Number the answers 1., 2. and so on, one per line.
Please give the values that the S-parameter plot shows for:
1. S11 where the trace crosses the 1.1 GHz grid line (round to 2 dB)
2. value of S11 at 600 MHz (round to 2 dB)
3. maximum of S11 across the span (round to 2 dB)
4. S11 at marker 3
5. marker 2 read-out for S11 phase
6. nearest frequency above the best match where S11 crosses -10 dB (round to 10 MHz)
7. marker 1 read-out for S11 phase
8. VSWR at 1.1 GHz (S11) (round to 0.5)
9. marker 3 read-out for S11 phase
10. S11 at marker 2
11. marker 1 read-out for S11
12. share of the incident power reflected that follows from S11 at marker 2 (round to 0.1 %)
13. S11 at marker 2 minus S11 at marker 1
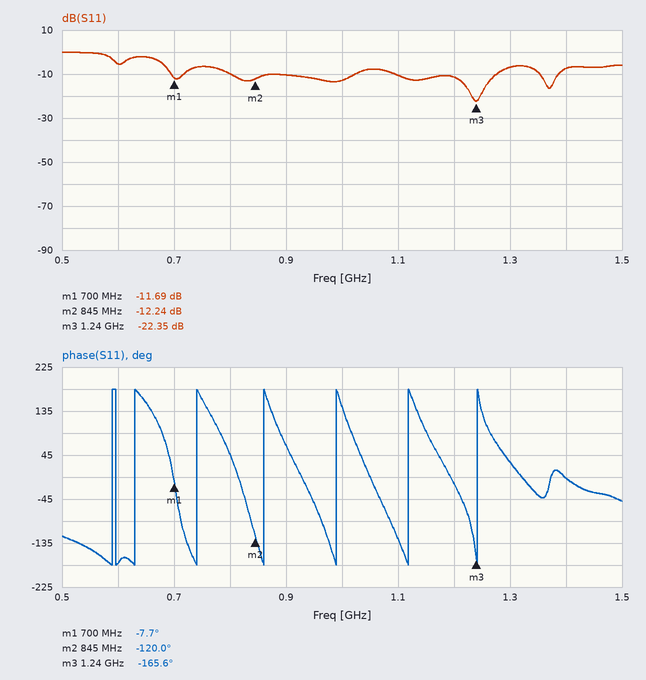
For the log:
1. -10 dB
2. -6 dB
3. 0 dB
4. -22.35 dB
5. -120.0°
6. 1.28 GHz
7. -7.7°
8. 2.0
9. -165.6°
10. -12.24 dB
11. -11.69 dB
12. 6.0 %
13. -0.55 dB
